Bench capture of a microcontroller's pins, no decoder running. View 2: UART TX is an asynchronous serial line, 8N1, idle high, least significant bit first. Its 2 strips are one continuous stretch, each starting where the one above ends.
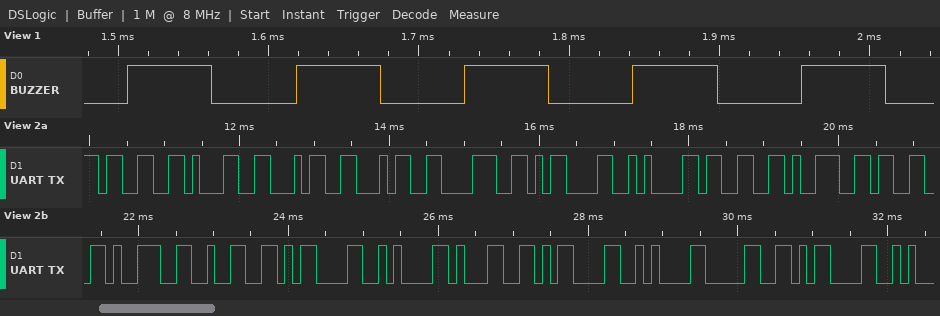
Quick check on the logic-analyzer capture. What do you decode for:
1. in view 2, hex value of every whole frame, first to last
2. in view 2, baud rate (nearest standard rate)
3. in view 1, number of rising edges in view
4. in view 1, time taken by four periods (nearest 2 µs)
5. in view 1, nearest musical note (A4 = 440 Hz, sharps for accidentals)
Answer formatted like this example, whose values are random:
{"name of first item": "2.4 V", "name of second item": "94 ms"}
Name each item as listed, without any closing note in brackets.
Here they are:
{"in view 2, hex value of every whole frame, first to last": "33 31 34 34 38 0D 0A 33 39 33 39 32 0D 0A 31 0D 0A 30 0D", "in view 2, baud rate": "9600 baud", "in view 1, number of rising edges in view": "5", "in view 1, time taken by four periods": "448 µs", "in view 1, nearest musical note": "C#9"}
